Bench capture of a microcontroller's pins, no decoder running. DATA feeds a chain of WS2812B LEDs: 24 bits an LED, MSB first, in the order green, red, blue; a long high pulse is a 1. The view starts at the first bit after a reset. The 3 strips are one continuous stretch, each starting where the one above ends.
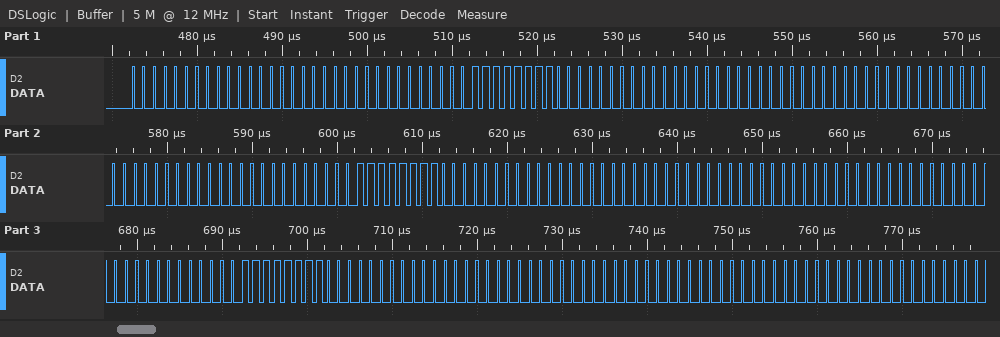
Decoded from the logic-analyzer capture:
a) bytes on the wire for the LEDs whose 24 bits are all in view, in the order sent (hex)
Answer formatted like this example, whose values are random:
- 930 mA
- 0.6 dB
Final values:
- 00 00 00 00 FF 00 00 00 00 00 00 00 00 FF 00 00 00 00 00 00 00 00 FF 00 00 00 00 00 00 00
